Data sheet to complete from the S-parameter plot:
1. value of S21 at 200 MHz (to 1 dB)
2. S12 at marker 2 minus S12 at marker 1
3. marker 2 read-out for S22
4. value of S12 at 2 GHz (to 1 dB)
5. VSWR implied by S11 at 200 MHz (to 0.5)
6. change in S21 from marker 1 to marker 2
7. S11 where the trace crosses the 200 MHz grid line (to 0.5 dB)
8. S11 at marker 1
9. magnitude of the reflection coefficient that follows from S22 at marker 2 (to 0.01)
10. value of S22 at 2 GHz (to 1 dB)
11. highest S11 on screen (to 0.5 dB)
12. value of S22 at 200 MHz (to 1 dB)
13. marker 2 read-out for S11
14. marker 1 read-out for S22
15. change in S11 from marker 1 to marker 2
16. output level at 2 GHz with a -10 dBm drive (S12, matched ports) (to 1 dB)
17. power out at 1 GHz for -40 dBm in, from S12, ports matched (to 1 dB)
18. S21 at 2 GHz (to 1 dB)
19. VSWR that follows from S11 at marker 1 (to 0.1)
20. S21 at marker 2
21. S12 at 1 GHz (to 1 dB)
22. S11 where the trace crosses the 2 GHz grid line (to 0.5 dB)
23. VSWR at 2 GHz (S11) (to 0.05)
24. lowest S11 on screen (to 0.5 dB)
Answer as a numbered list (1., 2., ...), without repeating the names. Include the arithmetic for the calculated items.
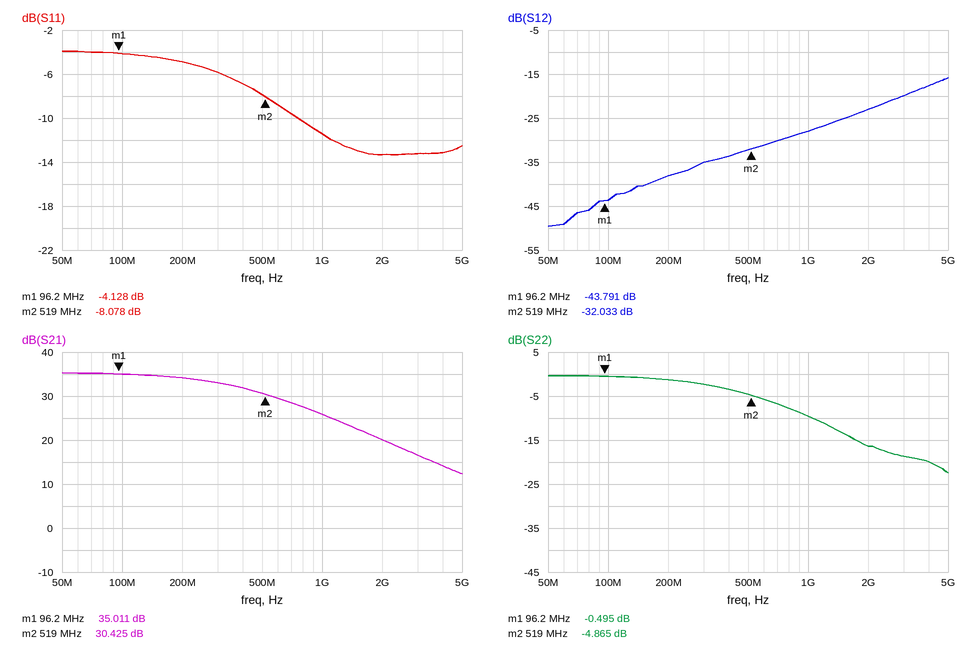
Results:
1. 34 dB
2. -32.033 − (-43.791) = 11.758 dB
3. -4.865 dB
4. -23 dB
5. |Γ| = 10^(-5/20) = 0.5623; VSWR = (1 + 0.5623)/(1 − 0.5623) ≈ 3.57, so 3.5 to the nearest 0.5
6. 30.425 − (35.011) = -4.586 dB
7. -5.0 dB
8. -4.128 dB
9. 10^(-4.865/20) ≈ 0.57
10. -16 dB
11. -4.0 dB
12. -1 dB
13. -8.078 dB
14. -0.495 dB
15. -8.078 − (-4.128) = -3.950 dB
16. -10 dBm + (-23 dB) = -33 dBm
17. -40 dBm + (-28 dB) = -68 dBm
18. 20 dB
19. (1 + 0.6217)/(1 − 0.6217) ≈ 4.3
20. 30.425 dB
21. -28 dB
22. -13.5 dB
23. |Γ| = 10^(-13.5/20) = 0.2113; VSWR = (1 + 0.2113)/(1 − 0.2113) ≈ 1.54, so 1.55 to the nearest 0.05
24. -13.5 dB
